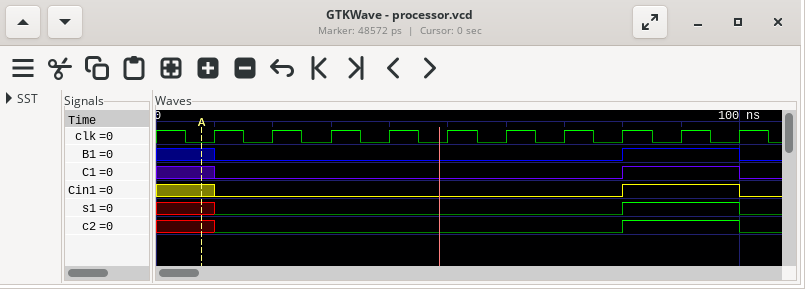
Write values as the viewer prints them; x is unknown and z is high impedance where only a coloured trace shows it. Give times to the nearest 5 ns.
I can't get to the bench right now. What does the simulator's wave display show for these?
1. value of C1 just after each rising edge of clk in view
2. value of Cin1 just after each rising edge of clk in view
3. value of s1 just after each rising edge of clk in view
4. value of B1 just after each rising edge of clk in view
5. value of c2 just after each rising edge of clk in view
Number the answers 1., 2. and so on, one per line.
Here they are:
1. 0 0 0 0 0 0 0 1 1 0
2. 0 0 0 0 0 0 0 1 1 0
3. 0 0 0 0 0 0 0 1 1 0
4. 0 0 0 0 0 0 0 1 1 0
5. 0 0 0 0 0 0 0 1 1 0
